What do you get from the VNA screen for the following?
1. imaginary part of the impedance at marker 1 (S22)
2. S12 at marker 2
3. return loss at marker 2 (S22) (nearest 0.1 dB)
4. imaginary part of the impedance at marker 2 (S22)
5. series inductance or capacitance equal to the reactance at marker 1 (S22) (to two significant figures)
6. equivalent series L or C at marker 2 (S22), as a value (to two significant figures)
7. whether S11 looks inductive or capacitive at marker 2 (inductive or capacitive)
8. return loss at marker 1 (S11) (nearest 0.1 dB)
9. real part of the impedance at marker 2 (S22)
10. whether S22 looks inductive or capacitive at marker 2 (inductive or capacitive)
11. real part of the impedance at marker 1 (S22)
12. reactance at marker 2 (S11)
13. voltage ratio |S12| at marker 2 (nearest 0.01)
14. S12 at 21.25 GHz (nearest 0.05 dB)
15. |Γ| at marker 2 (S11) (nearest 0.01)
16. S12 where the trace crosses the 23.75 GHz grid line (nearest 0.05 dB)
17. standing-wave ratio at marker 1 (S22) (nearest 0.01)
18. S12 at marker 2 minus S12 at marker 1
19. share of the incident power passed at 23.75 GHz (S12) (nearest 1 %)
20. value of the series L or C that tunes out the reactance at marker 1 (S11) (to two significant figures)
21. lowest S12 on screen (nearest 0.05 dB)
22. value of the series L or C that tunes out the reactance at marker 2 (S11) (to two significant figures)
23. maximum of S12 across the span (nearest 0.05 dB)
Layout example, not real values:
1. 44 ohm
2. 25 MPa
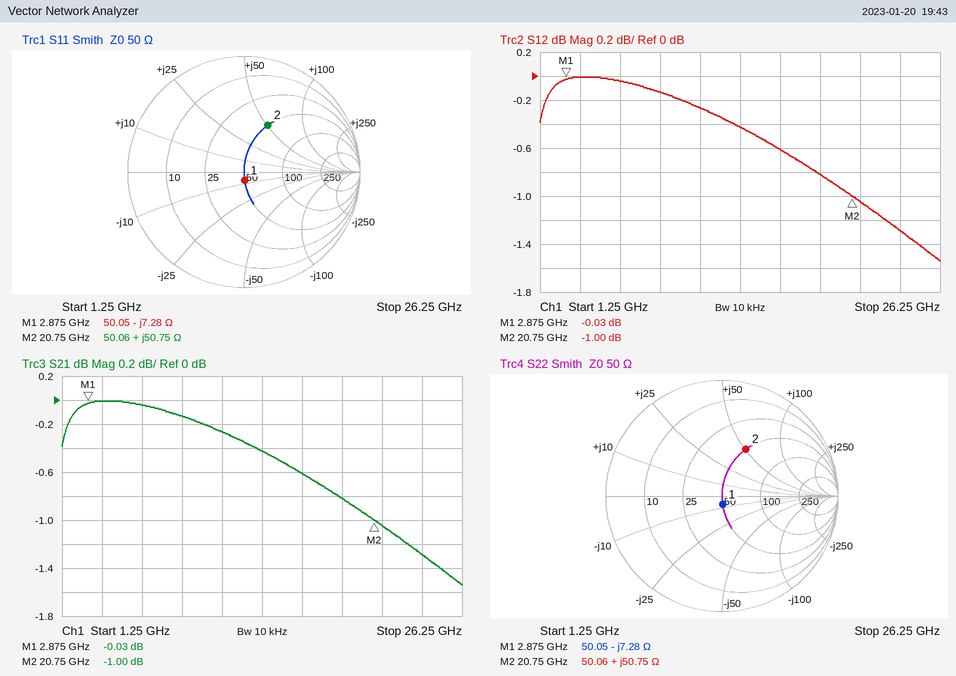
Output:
1. -7.28 Ω
2. -1.00 dB
3. 6.9 dB
4. +50.75 Ω
5. 7.6 pF
6. 390 pH
7. inductive
8. 22.8 dB
9. 50.06 Ω
10. inductive
11. 50.05 Ω
12. +50.75 Ω
13. 0.89
14. -1.05 dB
15. 0.45
16. -1.30 dB
17. 1.16
18. -0.97 dB
19. 74 %
20. 400 pH
21. -1.55 dB
22. 150 fF
23. 0.00 dB
